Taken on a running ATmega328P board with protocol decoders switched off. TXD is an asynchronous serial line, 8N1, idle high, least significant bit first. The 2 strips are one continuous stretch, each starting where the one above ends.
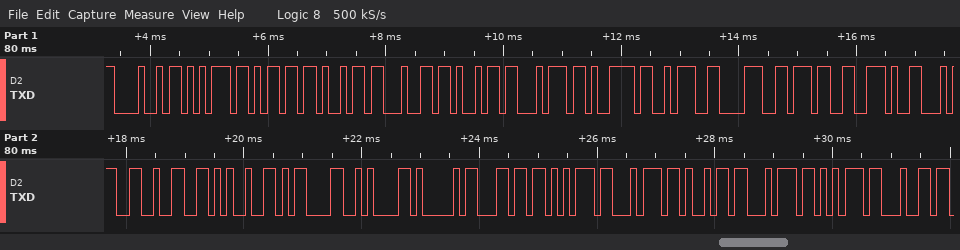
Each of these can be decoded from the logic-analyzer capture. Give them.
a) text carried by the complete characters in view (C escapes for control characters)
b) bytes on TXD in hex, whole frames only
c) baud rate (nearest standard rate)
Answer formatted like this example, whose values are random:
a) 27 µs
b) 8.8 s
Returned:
a) "Humidity:87.42%\r\nAlutitud"
b) 0x48 0x75 0x6D 0x69 0x64 0x69 0x74 0x79 0x3A 0x38 0x37 0x2E 0x34 0x32 0x25 0x0D 0x0A 0x41 0x6C 0x75 0x74 0x69 0x74 0x75 0x64
c) 9600 baud
